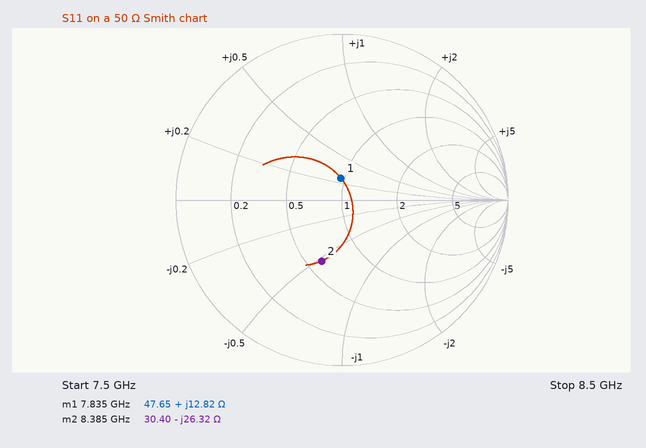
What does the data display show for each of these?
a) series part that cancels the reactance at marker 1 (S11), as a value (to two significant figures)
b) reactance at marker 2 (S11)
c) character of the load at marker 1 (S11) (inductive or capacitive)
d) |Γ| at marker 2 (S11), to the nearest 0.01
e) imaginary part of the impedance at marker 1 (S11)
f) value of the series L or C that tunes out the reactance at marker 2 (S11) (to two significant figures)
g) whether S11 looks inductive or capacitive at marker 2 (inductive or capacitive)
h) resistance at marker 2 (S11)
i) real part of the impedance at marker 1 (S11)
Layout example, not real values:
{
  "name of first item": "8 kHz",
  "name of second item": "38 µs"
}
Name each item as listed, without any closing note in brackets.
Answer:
{
  "series part that cancels the reactance at marker 1 (S11), as a value": "1.6 pF",
  "reactance at marker 2": "-26.32 Ω",
  "character of the load at marker 1 (S11)": "inductive",
  "|Γ| at marker 2 (S11), to the nearest 0.01": "0.39",
  "imaginary part of the impedance at marker 1": "+12.82 Ω",
  "value of the series L or C that tunes out the reactance at marker 2 (S11)": "500 pH",
  "whether S11 looks inductive or capacitive at marker 2": "capacitive",
  "resistance at marker 2": "30.40 Ω",
  "real part of the impedance at marker 1": "47.65 Ω"
}
